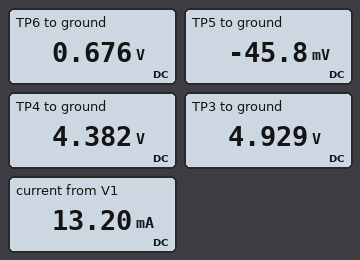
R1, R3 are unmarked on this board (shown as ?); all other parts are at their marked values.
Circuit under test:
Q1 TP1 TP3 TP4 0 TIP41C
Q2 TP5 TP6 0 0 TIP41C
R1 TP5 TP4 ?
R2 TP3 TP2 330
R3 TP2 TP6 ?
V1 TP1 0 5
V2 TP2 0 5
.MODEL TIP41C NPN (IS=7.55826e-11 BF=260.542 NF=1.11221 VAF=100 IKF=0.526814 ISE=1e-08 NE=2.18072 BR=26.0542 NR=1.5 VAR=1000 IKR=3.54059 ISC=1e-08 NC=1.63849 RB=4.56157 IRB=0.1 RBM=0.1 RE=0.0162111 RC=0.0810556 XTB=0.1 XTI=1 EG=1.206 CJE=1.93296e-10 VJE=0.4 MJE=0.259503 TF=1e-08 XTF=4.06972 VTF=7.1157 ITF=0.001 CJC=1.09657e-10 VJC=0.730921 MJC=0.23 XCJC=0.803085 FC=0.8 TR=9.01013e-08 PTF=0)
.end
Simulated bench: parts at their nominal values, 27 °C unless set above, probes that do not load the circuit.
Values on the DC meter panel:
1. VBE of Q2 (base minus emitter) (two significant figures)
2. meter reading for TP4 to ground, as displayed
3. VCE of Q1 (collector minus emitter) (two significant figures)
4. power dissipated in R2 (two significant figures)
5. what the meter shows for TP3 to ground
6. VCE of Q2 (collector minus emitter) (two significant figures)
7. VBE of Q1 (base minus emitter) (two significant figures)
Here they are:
680 mV
4.382 V
620 mV
15 µW
4.929 V
-46 mV
550 mV
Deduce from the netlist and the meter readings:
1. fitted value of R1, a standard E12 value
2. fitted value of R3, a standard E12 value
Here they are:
330 Ω
150 Ω
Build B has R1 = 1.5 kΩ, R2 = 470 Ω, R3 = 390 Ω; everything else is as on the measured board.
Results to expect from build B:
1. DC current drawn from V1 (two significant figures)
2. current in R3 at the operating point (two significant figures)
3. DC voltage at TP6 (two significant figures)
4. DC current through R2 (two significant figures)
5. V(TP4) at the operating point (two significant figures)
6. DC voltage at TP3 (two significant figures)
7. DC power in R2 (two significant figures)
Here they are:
2.9 mA
11 mA
590 mV
85 µA
4.5 V
5.0 V
3.4 µW
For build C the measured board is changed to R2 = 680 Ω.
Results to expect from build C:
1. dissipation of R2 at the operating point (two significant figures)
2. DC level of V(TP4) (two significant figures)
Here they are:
30 µW
4.3 V
